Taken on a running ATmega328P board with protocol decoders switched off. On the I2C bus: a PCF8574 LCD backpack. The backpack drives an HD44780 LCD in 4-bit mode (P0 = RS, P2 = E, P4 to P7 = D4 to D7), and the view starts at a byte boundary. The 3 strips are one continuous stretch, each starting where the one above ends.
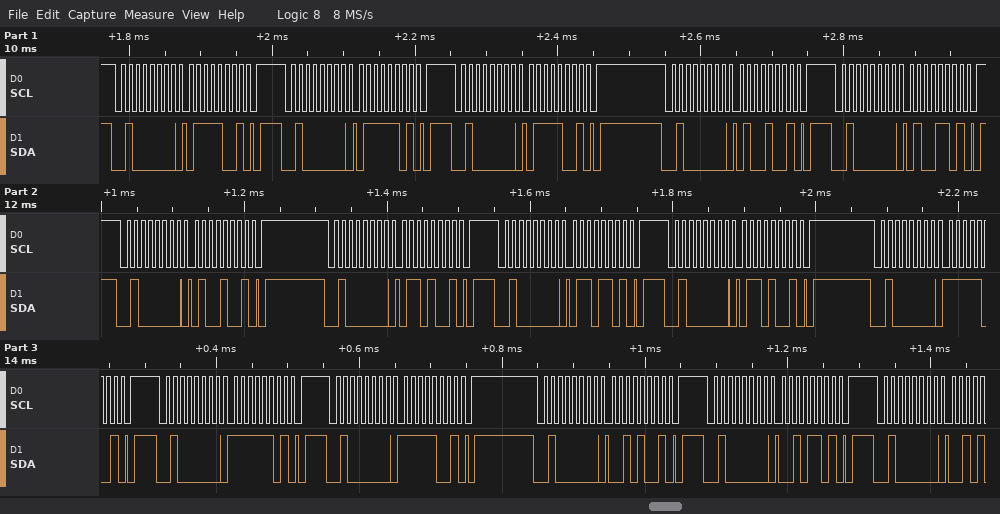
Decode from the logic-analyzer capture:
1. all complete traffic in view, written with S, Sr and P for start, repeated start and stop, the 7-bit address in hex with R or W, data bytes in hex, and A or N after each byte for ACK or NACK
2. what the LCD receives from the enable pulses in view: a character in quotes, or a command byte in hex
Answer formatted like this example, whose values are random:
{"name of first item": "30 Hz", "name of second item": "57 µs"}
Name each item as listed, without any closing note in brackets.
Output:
{"all complete traffic in view, written with S, Sr and P for start, repeated start and stop, the 7-bit address in hex with R or W, data bytes in hex, and A or N after each byte for ACK or NACK": "S 20W A 79 A P S 20W A 7D A P S 20W A 79 A P S 20W A 49 A P S 20W A 4D A P S 20W A 49 A P S 20W A 69 A P S 20W A 6D A P S 20W A 69 A P S 20W A F9 A P S 20W A FD A P S 20W A F9 A P S 20W A 29 A P S 20W A 2D A P S 20W A", "what the LCD receives from the enable pulses in view: a character in quotes, or a command byte in hex": "'t' 'o'"}
